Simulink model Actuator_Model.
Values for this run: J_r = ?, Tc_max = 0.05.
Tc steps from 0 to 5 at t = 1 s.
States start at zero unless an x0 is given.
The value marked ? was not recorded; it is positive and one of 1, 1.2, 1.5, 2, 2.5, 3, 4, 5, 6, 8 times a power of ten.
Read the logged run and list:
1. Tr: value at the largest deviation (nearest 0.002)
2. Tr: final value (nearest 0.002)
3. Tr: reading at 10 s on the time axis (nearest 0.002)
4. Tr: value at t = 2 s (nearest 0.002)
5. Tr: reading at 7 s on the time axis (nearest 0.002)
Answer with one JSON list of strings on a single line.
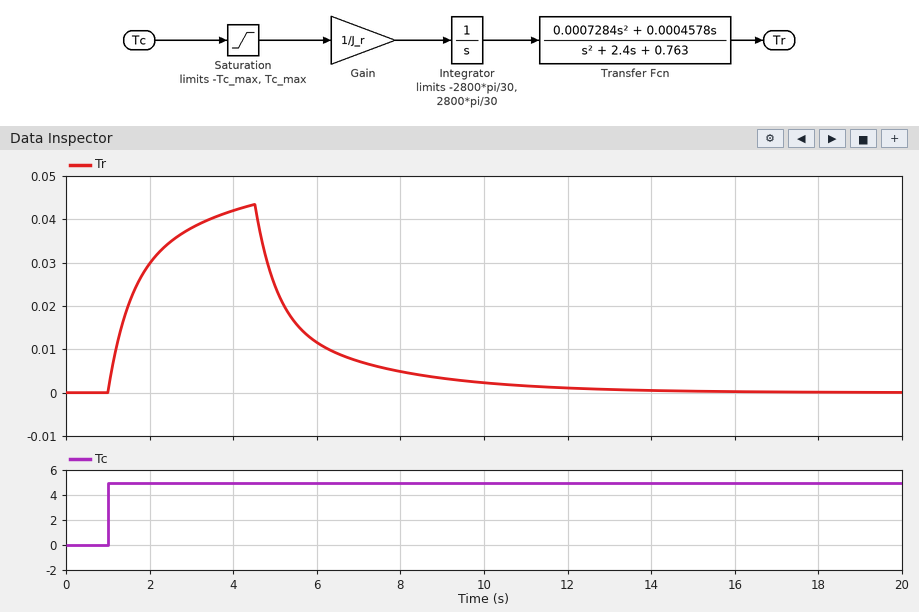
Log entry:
["0.044", "0.000", "0.002", "0.030", "0.008"]
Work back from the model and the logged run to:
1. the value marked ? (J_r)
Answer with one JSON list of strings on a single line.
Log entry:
["0.0006"]
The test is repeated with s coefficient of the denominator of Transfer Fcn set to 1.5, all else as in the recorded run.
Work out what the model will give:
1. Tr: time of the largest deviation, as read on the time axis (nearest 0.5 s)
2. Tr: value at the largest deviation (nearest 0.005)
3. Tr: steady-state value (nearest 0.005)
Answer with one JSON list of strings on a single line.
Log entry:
["4.0 s", "0.055", "0.000"]
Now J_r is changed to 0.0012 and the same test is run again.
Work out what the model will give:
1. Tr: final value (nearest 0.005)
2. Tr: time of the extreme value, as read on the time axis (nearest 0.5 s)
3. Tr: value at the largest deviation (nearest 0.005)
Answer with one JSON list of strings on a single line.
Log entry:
["0.000", "8.0 s", "0.050"]
